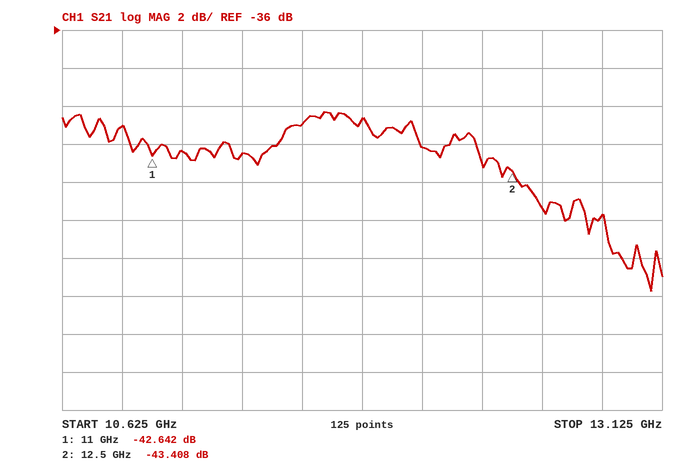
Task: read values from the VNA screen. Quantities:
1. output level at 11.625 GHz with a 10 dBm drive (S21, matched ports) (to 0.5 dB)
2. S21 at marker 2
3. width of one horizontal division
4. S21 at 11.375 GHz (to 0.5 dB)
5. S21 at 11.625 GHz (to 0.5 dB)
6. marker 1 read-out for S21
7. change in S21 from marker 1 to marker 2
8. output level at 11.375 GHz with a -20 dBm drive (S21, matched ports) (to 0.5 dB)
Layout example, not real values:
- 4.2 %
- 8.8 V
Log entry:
- -31.0 dBm
- -43.408 dB
- 250 MHz
- -42.5 dB
- -41.0 dB
- -42.642 dB
- -0.766 dB
- -62.5 dBm
